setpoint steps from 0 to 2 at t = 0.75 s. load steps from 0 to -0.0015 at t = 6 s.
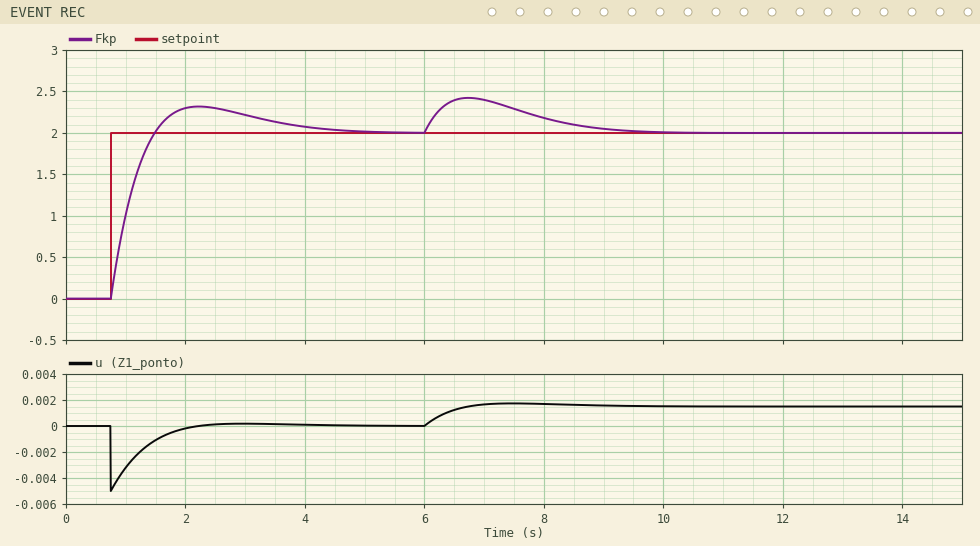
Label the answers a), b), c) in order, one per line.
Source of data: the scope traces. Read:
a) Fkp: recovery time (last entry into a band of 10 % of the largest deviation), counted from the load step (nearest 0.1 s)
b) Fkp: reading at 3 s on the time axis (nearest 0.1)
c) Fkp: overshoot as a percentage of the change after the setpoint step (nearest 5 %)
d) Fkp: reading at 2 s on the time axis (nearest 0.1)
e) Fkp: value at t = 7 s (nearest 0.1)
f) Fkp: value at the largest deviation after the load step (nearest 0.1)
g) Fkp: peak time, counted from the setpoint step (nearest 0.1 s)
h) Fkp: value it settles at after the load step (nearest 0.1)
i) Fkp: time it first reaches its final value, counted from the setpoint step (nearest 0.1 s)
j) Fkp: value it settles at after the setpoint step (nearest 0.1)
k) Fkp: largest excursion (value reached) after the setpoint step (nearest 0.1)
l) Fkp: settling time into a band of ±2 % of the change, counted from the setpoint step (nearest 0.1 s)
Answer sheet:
a) 3.1 s
b) 2.2
c) 15 %
d) 2.3
e) 2.4
f) 2.4
g) 1.5 s
h) 2.0
i) 0.7 s
j) 2.0
k) 2.3
l) 3.7 s
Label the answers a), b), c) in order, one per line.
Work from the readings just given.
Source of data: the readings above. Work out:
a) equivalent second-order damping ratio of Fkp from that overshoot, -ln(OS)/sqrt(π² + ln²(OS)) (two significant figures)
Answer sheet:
a) 0.52
